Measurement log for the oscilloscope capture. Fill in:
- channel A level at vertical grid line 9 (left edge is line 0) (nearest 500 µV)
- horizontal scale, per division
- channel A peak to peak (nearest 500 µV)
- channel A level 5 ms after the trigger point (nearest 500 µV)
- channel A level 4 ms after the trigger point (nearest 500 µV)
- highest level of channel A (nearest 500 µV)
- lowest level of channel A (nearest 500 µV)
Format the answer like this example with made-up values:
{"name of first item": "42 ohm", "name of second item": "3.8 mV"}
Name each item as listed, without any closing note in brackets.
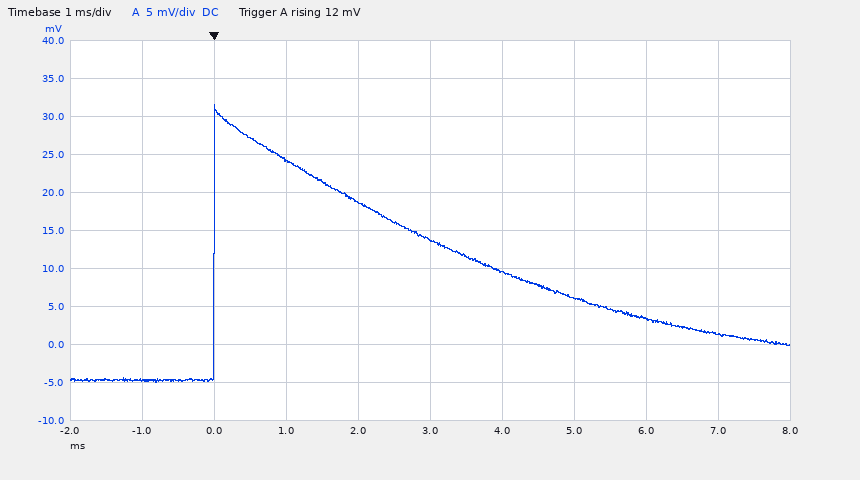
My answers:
{"channel A level at vertical grid line 9 (left edge is line 0)": "1.5 mV", "horizontal scale, per division": "1 ms", "channel A peak to peak": "36.5 mV", "channel A level 5 ms after the trigger point": "6.0 mV", "channel A level 4 ms after the trigger point": "9.5 mV", "highest level of channel A": "31.5 mV", "lowest level of channel A": "-5.0 mV"}
